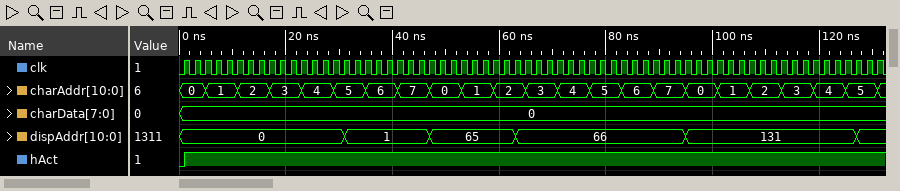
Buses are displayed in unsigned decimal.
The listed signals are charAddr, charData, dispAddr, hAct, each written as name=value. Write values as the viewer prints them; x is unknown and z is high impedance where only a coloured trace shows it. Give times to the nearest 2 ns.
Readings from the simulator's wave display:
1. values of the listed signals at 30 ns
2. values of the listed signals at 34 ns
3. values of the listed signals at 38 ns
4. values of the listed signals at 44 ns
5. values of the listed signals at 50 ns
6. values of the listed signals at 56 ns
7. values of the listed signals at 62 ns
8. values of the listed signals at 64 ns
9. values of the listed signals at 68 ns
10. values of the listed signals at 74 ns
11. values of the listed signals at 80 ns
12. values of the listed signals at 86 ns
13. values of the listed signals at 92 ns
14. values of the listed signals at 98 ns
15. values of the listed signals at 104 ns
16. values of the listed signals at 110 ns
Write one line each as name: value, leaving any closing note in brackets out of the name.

values of the listed signals at 30 ns: charAddr=5, charData=0, dispAddr=0, hAct=1
values of the listed signals at 34 ns: charAddr=5, charData=0, dispAddr=1, hAct=1
values of the listed signals at 38 ns: charAddr=6, charData=0, dispAddr=1, hAct=1
values of the listed signals at 44 ns: charAddr=7, charData=0, dispAddr=1, hAct=1
values of the listed signals at 50 ns: charAddr=0, charData=0, dispAddr=65, hAct=1
values of the listed signals at 56 ns: charAddr=1, charData=0, dispAddr=65, hAct=1
values of the listed signals at 62 ns: charAddr=2, charData=0, dispAddr=65, hAct=1
values of the listed signals at 64 ns: charAddr=2, charData=0, dispAddr=66, hAct=1
values of the listed signals at 68 ns: charAddr=3, charData=0, dispAddr=66, hAct=1
values of the listed signals at 74 ns: charAddr=4, charData=0, dispAddr=66, hAct=1
values of the listed signals at 80 ns: charAddr=5, charData=0, dispAddr=66, hAct=1
values of the listed signals at 86 ns: charAddr=6, charData=0, dispAddr=66, hAct=1
values of the listed signals at 92 ns: charAddr=7, charData=0, dispAddr=66, hAct=1
values of the listed signals at 98 ns: charAddr=0, charData=0, dispAddr=131, hAct=1
values of the listed signals at 104 ns: charAddr=1, charData=0, dispAddr=131, hAct=1
values of the listed signals at 110 ns: charAddr=2, charData=0, dispAddr=131, hAct=1
